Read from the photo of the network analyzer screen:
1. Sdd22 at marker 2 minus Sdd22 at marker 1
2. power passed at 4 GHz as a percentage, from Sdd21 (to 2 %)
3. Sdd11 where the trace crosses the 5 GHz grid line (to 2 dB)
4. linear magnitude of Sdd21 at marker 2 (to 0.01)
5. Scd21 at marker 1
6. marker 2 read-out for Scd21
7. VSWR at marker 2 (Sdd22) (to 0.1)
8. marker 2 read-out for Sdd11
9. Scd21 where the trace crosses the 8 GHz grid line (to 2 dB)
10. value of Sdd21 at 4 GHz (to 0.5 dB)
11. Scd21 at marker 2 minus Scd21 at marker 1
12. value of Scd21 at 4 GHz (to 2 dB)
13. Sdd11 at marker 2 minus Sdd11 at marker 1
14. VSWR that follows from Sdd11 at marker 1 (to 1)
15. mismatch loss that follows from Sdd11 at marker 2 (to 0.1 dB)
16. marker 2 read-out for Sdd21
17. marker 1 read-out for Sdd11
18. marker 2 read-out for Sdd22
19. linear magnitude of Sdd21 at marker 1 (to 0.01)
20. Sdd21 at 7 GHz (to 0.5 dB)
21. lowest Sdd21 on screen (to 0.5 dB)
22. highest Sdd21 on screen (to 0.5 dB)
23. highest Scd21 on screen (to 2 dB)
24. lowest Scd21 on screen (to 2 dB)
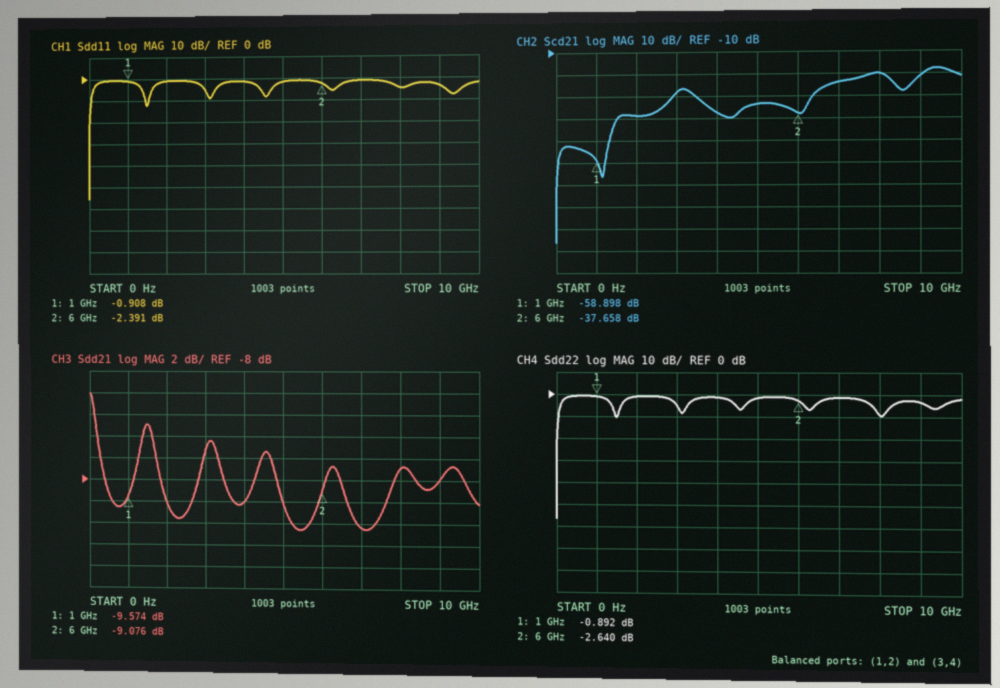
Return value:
-1.748 dB
10 %
-2 dB
0.35
-58.898 dB
-37.658 dB
6.6
-2.391 dB
-20 dB
-10.0 dB
21.240 dB
-38 dB
-1.483 dB
19
3.7 dB
-9.076 dB
-0.908 dB
-2.640 dB
0.33
-12.5 dB
-12.5 dB
0.0 dB
-18 dB
-96 dB
